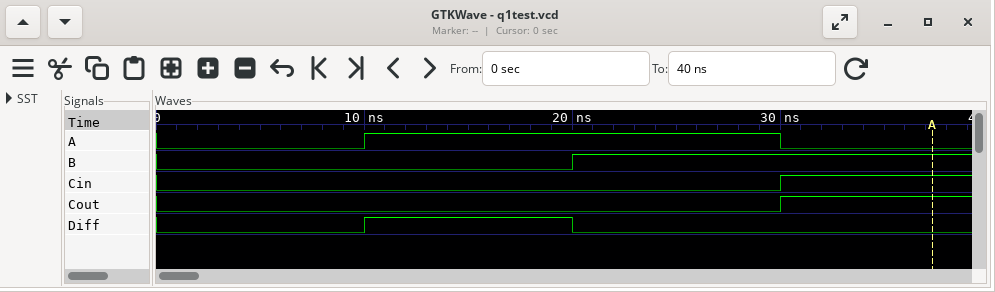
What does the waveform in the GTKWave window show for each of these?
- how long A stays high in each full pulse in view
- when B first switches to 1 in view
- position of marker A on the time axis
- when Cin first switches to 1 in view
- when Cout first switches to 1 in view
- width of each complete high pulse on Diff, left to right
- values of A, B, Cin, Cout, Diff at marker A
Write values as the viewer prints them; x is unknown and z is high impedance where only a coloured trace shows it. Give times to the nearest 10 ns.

20 ns
20 ns
40 ns
30 ns
30 ns
10 ns
A=0, B=1, Cin=1, Cout=1, Diff=0
